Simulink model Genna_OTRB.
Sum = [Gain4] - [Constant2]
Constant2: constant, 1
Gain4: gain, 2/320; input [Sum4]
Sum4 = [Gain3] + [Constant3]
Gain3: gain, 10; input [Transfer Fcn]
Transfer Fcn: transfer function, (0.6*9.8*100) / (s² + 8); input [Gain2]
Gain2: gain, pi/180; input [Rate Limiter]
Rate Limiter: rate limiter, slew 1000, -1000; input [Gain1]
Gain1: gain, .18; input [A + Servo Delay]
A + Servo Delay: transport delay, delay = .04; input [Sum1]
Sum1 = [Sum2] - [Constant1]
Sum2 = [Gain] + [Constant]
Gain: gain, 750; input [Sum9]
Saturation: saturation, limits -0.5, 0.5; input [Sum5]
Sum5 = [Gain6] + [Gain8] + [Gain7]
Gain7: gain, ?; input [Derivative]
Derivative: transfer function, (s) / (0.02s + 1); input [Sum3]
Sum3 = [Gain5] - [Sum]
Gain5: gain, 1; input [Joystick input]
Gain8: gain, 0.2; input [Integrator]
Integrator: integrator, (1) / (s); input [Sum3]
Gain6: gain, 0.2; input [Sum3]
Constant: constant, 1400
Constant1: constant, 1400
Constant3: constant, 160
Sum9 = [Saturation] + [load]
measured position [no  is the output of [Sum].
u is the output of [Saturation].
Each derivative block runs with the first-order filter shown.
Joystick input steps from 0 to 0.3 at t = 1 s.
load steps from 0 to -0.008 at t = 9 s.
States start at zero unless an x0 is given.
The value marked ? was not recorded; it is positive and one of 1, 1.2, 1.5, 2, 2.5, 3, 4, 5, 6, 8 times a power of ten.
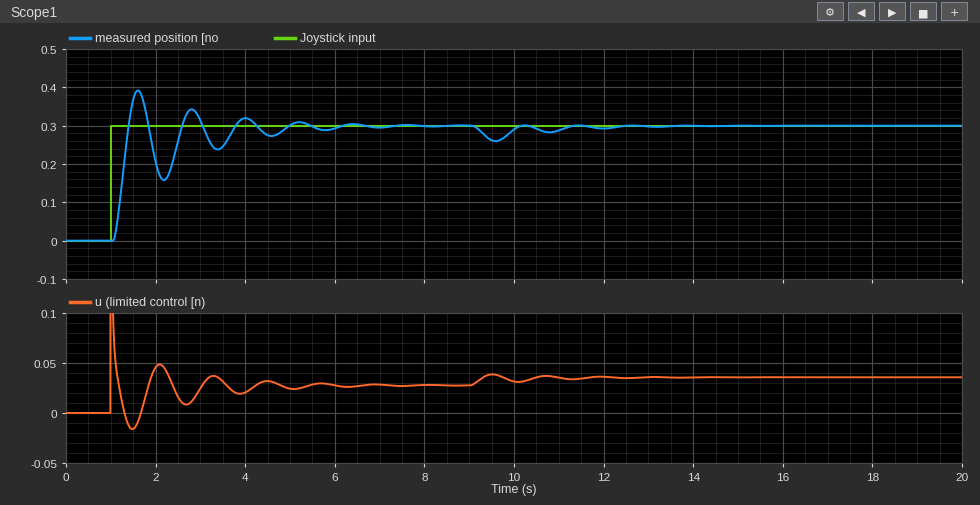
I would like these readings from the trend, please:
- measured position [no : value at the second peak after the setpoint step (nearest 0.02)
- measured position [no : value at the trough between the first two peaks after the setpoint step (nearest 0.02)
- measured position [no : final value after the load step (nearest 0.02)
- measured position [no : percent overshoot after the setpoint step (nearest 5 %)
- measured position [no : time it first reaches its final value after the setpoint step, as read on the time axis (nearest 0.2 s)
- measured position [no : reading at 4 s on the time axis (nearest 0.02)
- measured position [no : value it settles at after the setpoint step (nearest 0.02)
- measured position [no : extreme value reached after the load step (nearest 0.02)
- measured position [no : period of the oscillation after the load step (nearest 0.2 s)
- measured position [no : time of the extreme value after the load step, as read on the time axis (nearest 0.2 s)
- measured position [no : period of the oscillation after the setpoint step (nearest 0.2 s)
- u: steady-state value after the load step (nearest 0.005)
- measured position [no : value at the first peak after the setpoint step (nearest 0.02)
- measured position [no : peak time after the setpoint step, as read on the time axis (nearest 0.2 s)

0.34
0.16
0.30
30 %
1.4 s
0.32
0.30
0.26
1.2 s
9.6 s
1.2 s
0.035
0.40
1.6 s
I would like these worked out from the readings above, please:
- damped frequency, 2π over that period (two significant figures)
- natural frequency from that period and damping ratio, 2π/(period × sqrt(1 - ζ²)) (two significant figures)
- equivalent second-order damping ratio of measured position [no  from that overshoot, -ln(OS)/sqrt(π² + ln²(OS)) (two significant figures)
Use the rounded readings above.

5.2 rad/s
5.6 rad/s
0.36
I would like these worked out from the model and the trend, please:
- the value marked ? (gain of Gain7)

0.03
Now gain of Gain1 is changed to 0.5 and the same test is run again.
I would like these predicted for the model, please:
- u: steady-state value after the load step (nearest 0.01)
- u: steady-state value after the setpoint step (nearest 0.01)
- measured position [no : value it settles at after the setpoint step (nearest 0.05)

0.02
0.01
0.30
